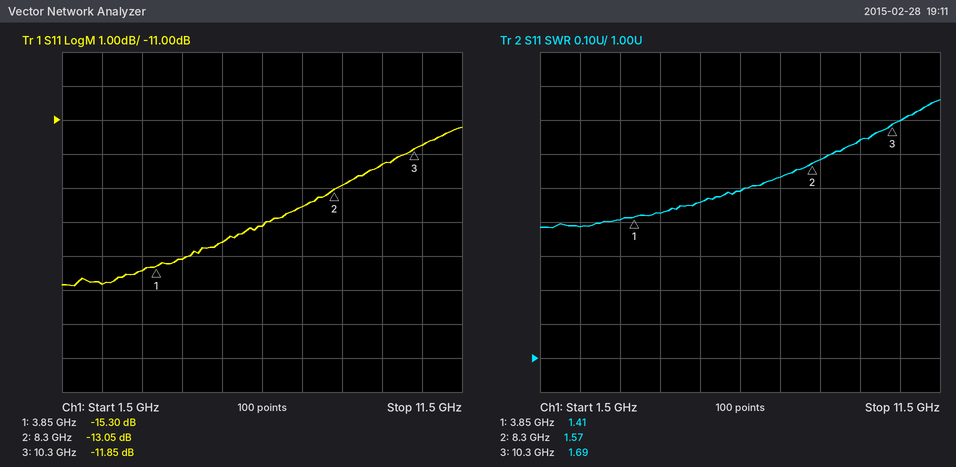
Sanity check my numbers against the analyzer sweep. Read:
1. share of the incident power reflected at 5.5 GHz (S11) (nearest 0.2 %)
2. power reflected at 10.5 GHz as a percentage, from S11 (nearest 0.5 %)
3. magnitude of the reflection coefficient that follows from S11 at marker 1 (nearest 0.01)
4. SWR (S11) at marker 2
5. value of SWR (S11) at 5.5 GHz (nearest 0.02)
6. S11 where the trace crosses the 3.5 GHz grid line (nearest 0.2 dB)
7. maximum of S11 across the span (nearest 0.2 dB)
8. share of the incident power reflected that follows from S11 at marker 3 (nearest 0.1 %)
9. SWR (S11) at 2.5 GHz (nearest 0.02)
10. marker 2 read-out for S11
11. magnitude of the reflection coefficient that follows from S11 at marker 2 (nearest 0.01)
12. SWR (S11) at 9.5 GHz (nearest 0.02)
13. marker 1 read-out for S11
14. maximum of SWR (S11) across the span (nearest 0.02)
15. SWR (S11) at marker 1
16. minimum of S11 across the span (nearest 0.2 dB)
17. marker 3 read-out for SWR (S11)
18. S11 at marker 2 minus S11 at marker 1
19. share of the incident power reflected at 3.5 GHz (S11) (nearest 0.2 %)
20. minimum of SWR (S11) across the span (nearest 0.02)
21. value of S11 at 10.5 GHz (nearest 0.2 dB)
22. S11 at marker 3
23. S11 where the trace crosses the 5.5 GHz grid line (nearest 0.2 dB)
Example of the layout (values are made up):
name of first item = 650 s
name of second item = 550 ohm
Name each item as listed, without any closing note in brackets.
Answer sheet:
share of the incident power reflected at 5.5 GHz (S11) = 3.4 %
power reflected at 10.5 GHz as a percentage, from S11 = 6.5 %
magnitude of the reflection coefficient that follows from S11 at marker 1 = 0.17
SWR (S11) at marker 2 = 1.57
value of SWR (S11) at 5.5 GHz = 1.46
S11 where the trace crosses the 3.5 GHz grid line = -15.4 dB
maximum of S11 across the span = -11.2 dB
share of the incident power reflected that follows from S11 at marker 3 = 6.5 %
SWR (S11) at 2.5 GHz = 1.38
marker 2 read-out for S11 = -13.05 dB
magnitude of the reflection coefficient that follows from S11 at marker 2 = 0.22
SWR (S11) at 9.5 GHz = 1.64
marker 1 read-out for S11 = -15.30 dB
maximum of SWR (S11) across the span = 1.76
SWR (S11) at marker 1 = 1.41
minimum of S11 across the span = -15.8 dB
marker 3 read-out for SWR = 1.69
S11 at marker 2 minus S11 at marker 1 = 2.25 dB
share of the incident power reflected at 3.5 GHz (S11) = 2.8 %
minimum of SWR (S11) across the span = 1.38
value of S11 at 10.5 GHz = -11.8 dB
S11 at marker 3 = -11.85 dB
S11 where the trace crosses the 5.5 GHz grid line = -14.6 dB
